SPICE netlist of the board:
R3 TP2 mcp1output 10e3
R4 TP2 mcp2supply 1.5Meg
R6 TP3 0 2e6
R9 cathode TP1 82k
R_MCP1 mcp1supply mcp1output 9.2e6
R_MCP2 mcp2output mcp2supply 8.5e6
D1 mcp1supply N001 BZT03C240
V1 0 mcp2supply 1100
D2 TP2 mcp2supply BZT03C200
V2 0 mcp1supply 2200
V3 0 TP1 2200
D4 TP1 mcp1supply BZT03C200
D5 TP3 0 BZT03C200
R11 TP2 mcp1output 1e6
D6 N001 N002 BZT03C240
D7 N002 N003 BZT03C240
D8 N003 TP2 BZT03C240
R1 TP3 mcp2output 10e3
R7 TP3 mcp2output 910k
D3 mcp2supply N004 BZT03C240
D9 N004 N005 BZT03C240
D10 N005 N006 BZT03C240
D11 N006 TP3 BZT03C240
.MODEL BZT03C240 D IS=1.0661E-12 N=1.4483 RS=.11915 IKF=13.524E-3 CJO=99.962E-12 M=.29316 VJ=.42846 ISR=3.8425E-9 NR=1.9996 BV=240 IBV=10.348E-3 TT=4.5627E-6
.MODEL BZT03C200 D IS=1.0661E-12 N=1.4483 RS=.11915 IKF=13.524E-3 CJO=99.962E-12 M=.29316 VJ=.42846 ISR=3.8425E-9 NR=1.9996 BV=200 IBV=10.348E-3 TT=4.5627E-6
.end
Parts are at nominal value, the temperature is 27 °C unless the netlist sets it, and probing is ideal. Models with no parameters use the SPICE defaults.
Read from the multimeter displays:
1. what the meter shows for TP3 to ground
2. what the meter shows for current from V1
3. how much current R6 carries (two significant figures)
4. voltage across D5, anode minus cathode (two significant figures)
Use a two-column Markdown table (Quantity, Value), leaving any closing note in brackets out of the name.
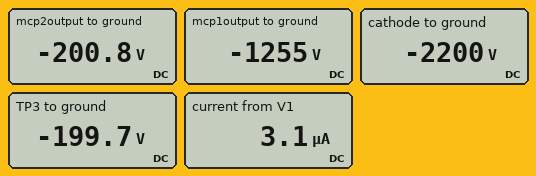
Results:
| Quantity | Value |
|---|---|
| what the meter shows for TP3 to ground | -199.7 V |
| what the meter shows for current from V1 | 3.1 µA |
| how much current R6 carries | 100 µA |
| voltage across D5, anode minus cathode | -200 V |
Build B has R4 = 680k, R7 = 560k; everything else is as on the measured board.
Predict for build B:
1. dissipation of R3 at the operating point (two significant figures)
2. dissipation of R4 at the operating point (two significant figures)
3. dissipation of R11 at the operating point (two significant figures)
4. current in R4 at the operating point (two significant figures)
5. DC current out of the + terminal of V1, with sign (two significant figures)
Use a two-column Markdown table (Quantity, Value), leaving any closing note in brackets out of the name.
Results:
| Quantity | Value |
|---|---|
| dissipation of R3 at the operating point | 110 µW |
| dissipation of R4 at the operating point | 29 mW |
| dissipation of R11 at the operating point | 1.1 µW |
| current in R4 at the operating point | 210 µA |
| DC current out of the + terminal of V1, with sign | -100 µA |
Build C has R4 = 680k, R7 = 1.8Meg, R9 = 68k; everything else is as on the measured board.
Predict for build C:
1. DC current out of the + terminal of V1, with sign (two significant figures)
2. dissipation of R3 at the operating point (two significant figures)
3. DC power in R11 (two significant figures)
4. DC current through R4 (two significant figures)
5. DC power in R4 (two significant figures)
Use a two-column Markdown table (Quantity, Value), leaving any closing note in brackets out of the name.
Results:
| Quantity | Value |
|---|---|
| DC current out of the + terminal of V1, with sign | -100 µA |
| dissipation of R3 at the operating point | 110 µW |
| DC power in R11 | 1.1 µW |
| DC current through R4 | 210 µA |
| DC power in R4 | 29 mW |
